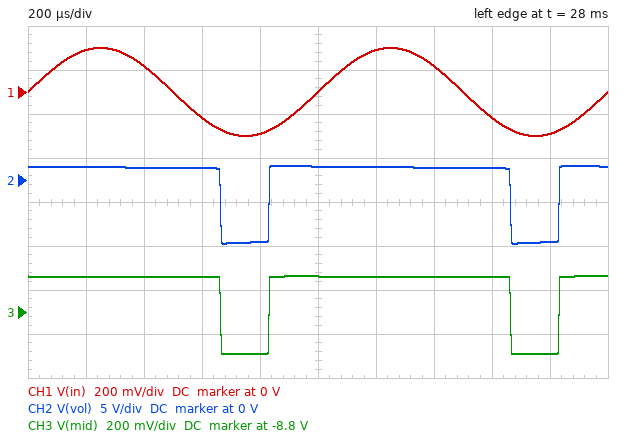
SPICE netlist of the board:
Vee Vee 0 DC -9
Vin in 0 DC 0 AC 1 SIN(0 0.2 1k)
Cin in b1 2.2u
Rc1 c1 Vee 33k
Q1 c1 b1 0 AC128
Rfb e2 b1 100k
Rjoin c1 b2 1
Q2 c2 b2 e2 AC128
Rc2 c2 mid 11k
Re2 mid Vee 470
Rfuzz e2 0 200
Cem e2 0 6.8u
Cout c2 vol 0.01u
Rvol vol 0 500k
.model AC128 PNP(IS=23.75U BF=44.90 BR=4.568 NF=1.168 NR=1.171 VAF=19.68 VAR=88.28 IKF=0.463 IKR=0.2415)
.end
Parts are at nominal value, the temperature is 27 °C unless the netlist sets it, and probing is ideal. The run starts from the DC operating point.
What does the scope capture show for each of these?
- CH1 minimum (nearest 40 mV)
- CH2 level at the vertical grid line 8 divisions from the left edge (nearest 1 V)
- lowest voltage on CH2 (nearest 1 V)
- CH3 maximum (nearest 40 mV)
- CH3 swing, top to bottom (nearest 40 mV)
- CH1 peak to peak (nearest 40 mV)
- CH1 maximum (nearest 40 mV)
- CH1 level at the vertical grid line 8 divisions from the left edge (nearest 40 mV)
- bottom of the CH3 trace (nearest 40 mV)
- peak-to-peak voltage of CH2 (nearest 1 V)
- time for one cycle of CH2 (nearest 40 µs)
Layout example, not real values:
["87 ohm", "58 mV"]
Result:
["-200 mV", "1 V", "-7 V", "-8.64 V", "360 mV", "400 mV", "200 mV", "-120 mV", "-9.00 V", "9 V", "1.00 ms"]
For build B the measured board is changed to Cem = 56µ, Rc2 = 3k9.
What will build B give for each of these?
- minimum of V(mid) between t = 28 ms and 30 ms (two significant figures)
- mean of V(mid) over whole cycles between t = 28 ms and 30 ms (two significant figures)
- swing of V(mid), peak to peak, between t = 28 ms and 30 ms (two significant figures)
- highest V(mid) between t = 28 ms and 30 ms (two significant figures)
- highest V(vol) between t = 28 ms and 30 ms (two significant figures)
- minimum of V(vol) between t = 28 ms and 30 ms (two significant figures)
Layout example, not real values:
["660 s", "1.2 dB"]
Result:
["-9.0 V", "-8.2 V", "920 mV", "-8.1 V", "1.7 V", "-7.1 V"]
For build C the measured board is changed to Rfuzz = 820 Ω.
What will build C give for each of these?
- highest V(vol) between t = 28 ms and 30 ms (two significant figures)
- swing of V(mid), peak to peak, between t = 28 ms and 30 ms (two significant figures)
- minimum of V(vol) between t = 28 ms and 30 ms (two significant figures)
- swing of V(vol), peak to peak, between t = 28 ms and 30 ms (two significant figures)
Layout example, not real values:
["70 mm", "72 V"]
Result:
["1.7 V", "330 mV", "-6.7 V", "8.4 V"]
